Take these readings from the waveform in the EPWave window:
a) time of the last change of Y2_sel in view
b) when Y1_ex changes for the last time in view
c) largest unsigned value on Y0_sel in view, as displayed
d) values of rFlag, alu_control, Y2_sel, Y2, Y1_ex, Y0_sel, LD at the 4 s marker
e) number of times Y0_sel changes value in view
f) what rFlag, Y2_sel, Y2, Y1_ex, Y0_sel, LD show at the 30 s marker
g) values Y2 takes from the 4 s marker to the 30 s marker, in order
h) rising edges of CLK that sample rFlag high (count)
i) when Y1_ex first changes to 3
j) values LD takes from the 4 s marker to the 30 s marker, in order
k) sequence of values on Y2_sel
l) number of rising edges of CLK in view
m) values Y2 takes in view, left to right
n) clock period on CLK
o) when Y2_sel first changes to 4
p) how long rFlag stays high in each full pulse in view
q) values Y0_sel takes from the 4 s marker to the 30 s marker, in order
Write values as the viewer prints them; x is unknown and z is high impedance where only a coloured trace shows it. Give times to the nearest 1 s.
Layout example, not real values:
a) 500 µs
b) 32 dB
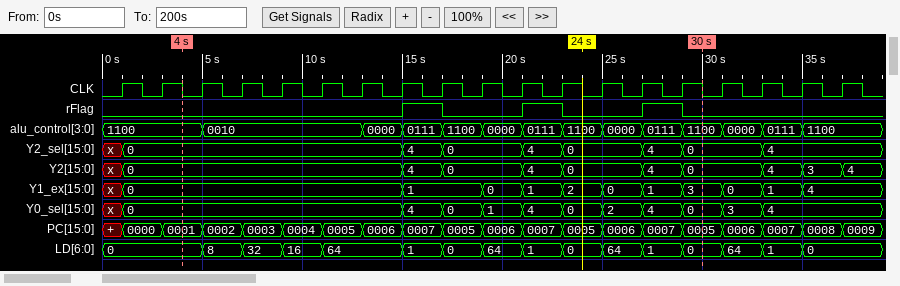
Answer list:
a) 33 s
b) 35 s
c) 4
d) rFlag=0, alu_control=1100, Y2_sel=0, Y2=0, Y1_ex=0, Y0_sel=0, LD=0
e) 11
f) rFlag=0, Y2_sel=0, Y2=0, Y1_ex=3, Y0_sel=0, LD=0
g) 0, 4, 0, 4, 0, 4, 0
h) 3
i) 29 s
j) 0, 8, 32, 16, 64, 1, 0, 64, 1, 0, 64, 1, 0
k) x, 0, 4, 0, 4, 0, 4, 0, 4
l) 19
m) x, 0, 4, 0, 4, 0, 4, 0, 4, 3, 4
n) 2 s
o) 15 s
p) 2 s, 2 s, 2 s
q) 0, 4, 0, 1, 4, 0, 2, 4, 0
